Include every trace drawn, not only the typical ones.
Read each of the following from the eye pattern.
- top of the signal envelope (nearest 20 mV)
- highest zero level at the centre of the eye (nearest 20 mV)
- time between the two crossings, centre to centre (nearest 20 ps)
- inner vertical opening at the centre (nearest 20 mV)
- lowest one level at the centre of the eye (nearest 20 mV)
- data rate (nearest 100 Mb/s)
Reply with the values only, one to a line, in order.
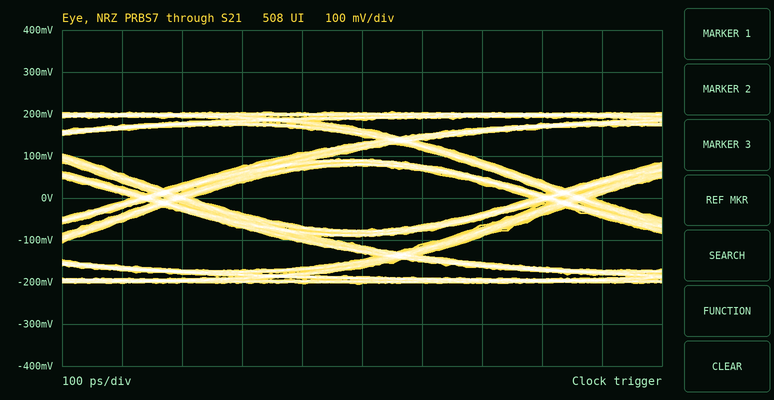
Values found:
200 mV
-80 mV
660 ps
160 mV
80 mV
1.5 Gb/s
